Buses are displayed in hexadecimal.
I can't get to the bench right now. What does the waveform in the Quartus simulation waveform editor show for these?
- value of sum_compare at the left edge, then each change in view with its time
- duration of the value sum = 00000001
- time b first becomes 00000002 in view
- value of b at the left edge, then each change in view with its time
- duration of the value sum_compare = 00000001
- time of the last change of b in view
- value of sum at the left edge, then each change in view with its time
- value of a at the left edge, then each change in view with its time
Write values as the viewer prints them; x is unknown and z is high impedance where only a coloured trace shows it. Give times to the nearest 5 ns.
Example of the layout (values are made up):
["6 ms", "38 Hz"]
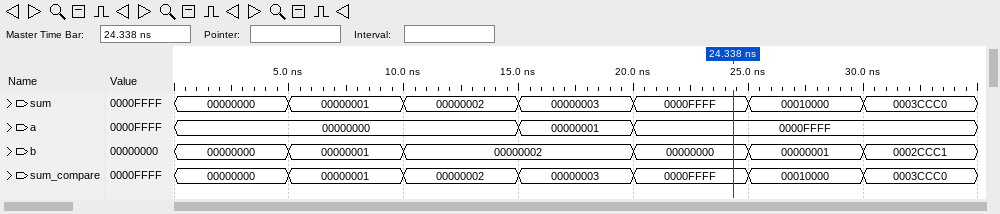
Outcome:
["00000000, 00000001 at 5 ns, 00000002 at 10 ns, 00000003 at 15 ns, 0000FFFF at 20 ns, 00010000 at 25 ns, 0003CCC0 at 30 ns", "5 ns", "10 ns", "00000000, 00000001 at 5 ns, 00000002 at 10 ns, 00000000 at 20 ns, 00000001 at 25 ns, 0002CCC1 at 30 ns", "5 ns", "30 ns", "00000000, 00000001 at 5 ns, 00000002 at 10 ns, 00000003 at 15 ns, 0000FFFF at 20 ns, 00010000 at 25 ns, 0003CCC0 at 30 ns", "00000000, 00000001 at 15 ns, 0000FFFF at 20 ns"]
